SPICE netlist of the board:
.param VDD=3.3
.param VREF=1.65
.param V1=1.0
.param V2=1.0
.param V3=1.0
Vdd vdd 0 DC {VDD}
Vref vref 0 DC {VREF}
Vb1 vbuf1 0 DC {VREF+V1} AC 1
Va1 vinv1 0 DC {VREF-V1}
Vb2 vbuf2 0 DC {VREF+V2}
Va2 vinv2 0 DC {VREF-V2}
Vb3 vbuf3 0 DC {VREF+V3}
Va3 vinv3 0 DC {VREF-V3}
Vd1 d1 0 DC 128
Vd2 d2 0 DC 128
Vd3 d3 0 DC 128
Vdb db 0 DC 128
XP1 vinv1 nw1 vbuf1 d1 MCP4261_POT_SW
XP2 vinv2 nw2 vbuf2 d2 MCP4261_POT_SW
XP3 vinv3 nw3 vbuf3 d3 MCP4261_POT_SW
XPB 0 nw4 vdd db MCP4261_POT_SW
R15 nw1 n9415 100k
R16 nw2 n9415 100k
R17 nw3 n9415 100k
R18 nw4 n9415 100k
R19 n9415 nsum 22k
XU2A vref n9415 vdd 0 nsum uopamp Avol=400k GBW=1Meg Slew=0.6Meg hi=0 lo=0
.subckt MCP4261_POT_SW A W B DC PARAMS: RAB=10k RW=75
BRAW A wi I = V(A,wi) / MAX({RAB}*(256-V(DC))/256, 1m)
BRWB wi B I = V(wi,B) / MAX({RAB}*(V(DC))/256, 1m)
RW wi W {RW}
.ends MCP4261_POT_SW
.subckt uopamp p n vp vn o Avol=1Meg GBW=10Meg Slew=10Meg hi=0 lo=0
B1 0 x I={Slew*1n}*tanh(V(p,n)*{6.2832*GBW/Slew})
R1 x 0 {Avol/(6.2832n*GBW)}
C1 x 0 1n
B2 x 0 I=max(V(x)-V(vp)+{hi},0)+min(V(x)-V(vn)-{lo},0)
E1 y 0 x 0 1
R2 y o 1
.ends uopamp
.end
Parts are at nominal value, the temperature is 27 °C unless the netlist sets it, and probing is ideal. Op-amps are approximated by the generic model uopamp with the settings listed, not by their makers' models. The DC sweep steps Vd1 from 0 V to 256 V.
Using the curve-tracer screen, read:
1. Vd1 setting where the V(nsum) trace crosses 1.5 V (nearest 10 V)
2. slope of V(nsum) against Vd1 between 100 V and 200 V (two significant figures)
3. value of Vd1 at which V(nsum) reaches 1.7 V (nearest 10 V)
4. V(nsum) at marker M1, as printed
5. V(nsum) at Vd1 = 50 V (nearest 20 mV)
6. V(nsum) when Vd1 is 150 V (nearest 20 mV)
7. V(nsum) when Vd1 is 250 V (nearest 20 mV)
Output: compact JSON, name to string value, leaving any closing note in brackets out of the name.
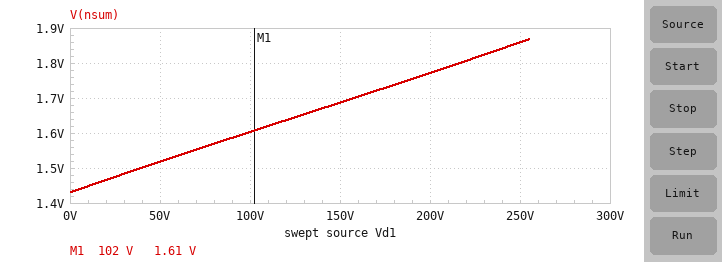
{"Vd1 setting where the V(nsum) trace crosses 1.5 V": "40 V", "slope of V(nsum) against Vd1 between 100 V and 200 V": "0.0017 V/V", "value of Vd1 at which V(nsum) reaches 1.7 V": "160 V", "V(nsum) at marker M1, as printed": "1.61 V", "V(nsum) at Vd1 = 50 V": "1.52 V", "V(nsum) when Vd1 is 150 V": "1.68 V", "V(nsum) when Vd1 is 250 V": "1.86 V"}
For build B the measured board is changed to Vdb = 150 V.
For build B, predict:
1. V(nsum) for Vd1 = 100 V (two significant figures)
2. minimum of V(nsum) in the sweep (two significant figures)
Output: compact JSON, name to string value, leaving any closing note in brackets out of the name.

{"V(nsum) for Vd1 = 100 V": "1.7 V", "minimum of V(nsum) in the sweep": "1.5 V"}
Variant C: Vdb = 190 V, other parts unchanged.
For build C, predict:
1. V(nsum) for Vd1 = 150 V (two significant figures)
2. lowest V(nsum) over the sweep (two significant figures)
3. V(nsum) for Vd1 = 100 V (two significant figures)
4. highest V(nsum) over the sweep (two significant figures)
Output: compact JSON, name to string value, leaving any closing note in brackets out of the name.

{"V(nsum) for Vd1 = 150 V": "1.9 V", "lowest V(nsum) over the sweep": "1.6 V", "V(nsum) for Vd1 = 100 V": "1.8 V", "highest V(nsum) over the sweep": "2.0 V"}
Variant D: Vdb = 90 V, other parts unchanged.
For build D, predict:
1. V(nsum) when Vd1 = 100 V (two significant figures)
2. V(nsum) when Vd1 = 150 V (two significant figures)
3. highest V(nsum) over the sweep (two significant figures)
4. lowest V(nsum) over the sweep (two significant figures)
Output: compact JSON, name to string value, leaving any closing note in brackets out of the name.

{"V(nsum) when Vd1 = 100 V": "1.5 V", "V(nsum) when Vd1 = 150 V": "1.6 V", "highest V(nsum) over the sweep": "1.8 V", "lowest V(nsum) over the sweep": "1.3 V"}
